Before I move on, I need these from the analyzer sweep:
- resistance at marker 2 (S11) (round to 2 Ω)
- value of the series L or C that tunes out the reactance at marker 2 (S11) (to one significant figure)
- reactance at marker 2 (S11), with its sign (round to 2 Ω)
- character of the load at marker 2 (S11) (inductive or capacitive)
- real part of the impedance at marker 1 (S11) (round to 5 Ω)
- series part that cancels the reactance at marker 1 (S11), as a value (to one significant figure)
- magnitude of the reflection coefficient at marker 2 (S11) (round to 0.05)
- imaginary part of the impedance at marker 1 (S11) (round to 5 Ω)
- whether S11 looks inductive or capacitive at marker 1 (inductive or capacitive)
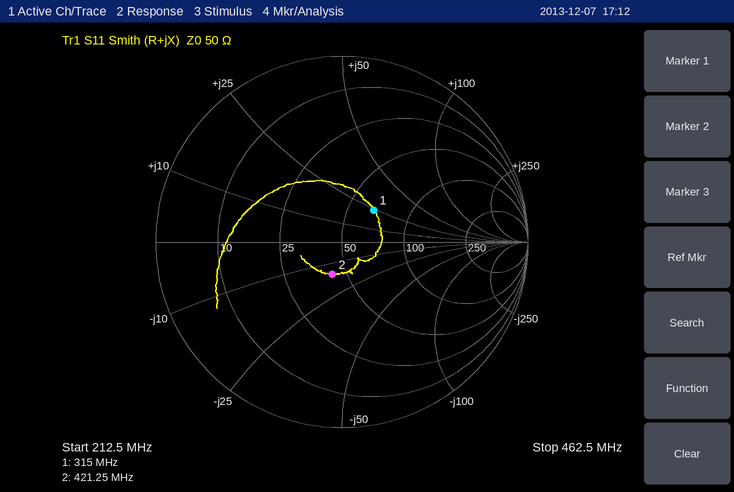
42 Ω
6 nH
-16 Ω
capacitive
65 Ω
20 pF
0.20
+25 Ω
inductive
